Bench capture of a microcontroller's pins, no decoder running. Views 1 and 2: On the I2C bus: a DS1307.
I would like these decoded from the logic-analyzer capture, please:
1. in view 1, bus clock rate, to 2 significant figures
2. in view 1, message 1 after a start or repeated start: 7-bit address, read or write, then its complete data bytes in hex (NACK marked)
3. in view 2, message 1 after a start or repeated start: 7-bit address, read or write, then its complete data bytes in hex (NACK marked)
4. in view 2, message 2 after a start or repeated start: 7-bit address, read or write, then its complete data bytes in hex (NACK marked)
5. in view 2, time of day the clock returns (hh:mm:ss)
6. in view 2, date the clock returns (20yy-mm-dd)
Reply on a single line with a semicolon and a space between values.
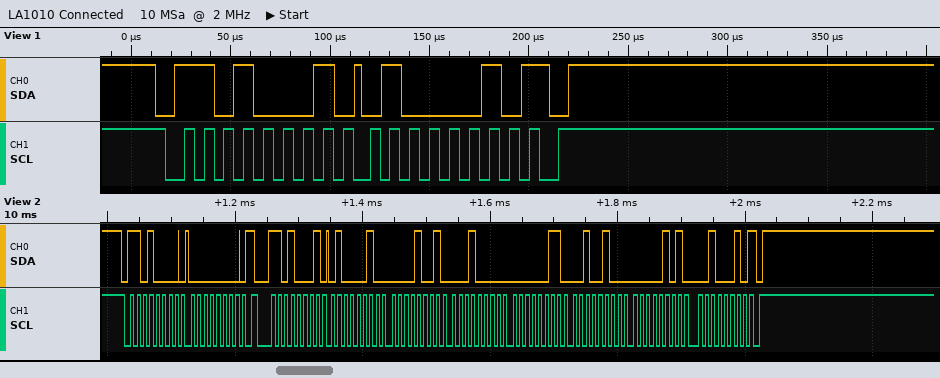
100 kHz; 0x68 read: 42 NACK; 0x68 write: 00; 0x68 read: 42 09 10 03 24 05 22 NACK; 10:09:42; 2022-05-24
